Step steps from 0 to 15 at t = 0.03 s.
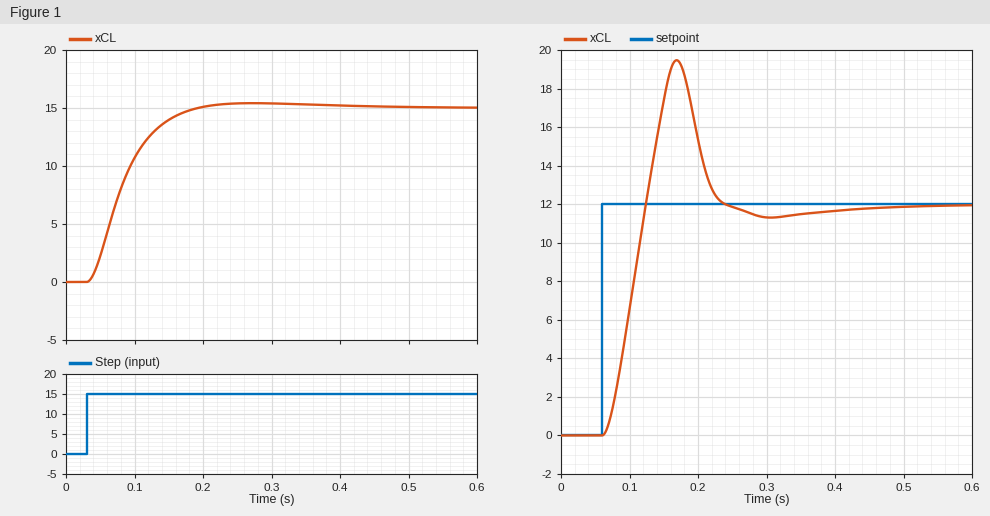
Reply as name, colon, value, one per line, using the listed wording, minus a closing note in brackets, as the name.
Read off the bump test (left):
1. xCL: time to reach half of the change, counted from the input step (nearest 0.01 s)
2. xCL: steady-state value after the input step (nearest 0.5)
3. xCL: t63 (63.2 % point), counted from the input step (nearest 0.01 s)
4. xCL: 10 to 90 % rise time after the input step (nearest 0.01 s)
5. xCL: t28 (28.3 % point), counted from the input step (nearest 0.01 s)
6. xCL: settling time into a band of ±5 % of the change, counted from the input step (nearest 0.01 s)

xCL: time to reach half of the change, counted from the input step: 0.05 s
xCL: steady-state value after the input step: 15.0
xCL: t63 (63.2 % point), counted from the input step: 0.06 s
xCL: 10 to 90 % rise time after the input step: 0.09 s
xCL: t28 (28.3 % point), counted from the input step: 0.03 s
xCL: settling time into a band of ±5 % of the change, counted from the input step: 0.13 s
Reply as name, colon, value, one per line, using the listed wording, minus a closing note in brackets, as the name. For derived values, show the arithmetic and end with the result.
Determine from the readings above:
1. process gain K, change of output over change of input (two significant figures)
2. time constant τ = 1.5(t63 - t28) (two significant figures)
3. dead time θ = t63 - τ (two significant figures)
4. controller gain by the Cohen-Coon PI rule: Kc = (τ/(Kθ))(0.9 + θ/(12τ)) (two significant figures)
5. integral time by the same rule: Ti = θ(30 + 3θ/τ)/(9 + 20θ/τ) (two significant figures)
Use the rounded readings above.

process gain K, change of output over change of input: (15 - 0) / 15 = 1.0
time constant τ = 1.5(t63 - t28): 1.5 × (0.06 - 0.03) = 0.045 s
dead time θ = t63 - τ: 0.06 - 0.045 = 0.015 s
controller gain by the Cohen-Coon PI rule: Kc = (τ/(Kθ))(0.9 + θ/(12τ)): 0.045 / (1 × 0.015) × (0.9 + 0.015 / (12 × 0.045)) = 2.8
integral time by the same rule: Ti = θ(30 + 3θ/τ)/(9 + 20θ/τ): 0.015 × (30 + 3 × 0.015 / 0.045) / (9 + 20 × 0.015 / 0.045) = 0.030 s
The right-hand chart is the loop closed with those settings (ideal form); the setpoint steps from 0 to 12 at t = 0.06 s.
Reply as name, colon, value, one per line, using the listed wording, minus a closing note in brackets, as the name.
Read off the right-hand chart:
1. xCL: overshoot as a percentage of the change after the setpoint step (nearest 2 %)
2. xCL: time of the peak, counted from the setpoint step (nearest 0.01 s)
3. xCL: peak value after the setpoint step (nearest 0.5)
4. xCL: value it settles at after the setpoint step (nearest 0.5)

xCL: overshoot as a percentage of the change after the setpoint step: 62 %
xCL: time of the peak, counted from the setpoint step: 0.11 s
xCL: peak value after the setpoint step: 19.5
xCL: value it settles at after the setpoint step: 12.0
